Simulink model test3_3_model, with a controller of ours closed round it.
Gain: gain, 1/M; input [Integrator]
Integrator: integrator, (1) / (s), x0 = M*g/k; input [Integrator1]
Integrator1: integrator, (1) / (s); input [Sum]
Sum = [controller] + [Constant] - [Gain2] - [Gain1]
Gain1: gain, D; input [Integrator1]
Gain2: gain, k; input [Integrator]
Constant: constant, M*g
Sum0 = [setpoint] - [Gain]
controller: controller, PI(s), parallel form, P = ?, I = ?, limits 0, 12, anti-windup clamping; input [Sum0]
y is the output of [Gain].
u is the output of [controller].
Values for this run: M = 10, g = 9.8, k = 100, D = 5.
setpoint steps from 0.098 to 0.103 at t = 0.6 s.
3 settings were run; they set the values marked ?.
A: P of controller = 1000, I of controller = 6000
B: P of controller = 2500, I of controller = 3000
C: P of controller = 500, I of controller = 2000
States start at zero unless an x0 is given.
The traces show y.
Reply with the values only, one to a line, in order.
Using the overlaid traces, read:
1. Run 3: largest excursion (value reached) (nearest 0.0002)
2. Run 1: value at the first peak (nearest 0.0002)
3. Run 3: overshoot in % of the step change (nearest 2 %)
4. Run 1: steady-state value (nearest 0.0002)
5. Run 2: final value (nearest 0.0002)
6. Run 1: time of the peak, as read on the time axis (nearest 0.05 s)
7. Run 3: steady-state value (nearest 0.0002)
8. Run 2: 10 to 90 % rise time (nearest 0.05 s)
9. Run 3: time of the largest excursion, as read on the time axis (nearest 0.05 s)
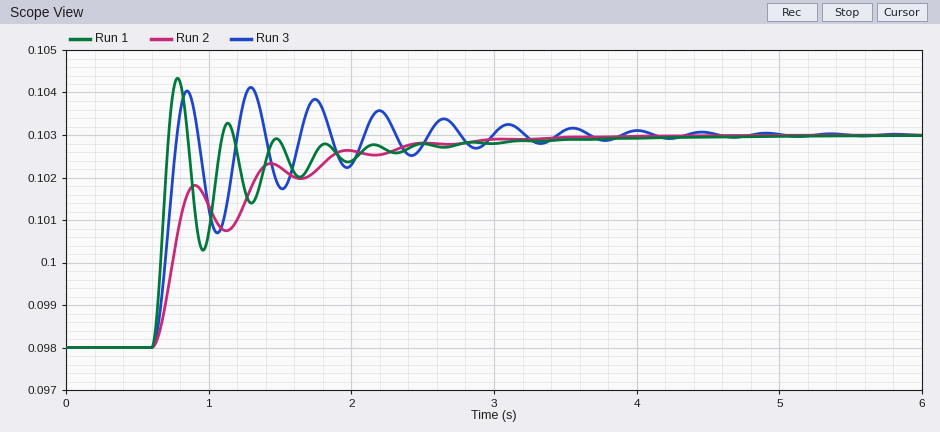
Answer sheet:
0.1042
0.1044
22 %
0.1030
0.1030
0.80 s
0.1030
1.20 s
1.30 s
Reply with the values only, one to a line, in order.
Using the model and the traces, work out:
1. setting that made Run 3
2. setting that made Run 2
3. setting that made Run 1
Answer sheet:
A
C
B
